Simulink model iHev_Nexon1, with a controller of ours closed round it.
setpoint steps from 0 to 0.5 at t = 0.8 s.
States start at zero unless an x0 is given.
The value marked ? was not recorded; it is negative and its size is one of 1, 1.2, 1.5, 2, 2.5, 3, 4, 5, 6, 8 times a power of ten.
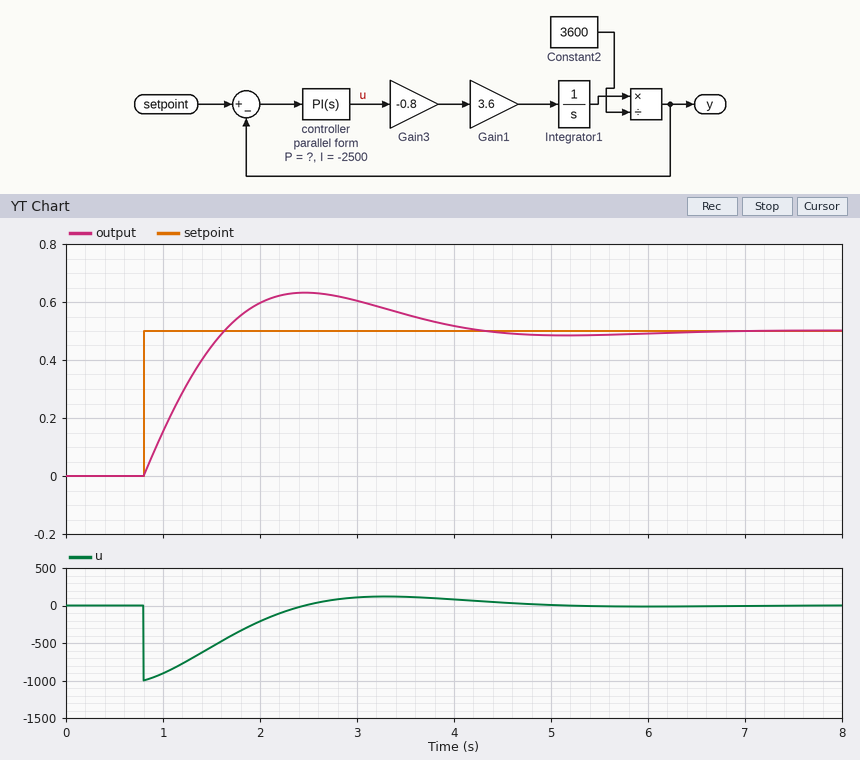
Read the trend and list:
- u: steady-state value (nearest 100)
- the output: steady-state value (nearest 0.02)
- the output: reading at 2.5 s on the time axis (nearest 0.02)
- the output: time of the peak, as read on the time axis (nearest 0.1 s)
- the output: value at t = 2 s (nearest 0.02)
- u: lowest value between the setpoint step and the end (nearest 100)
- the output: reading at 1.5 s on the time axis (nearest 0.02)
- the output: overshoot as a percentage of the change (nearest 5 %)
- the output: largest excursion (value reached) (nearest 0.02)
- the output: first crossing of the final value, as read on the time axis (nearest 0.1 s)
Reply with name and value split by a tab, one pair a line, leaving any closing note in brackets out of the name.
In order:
u: steady-state value	0
the output: steady-state value	0.50
the output: reading at 2.5 s on the time axis	0.64
the output: time of the peak, as read on the time axis	2.5 s
the output: value at t = 2 s	0.60
u: lowest value between the setpoint step and the end	-1000
the output: reading at 1.5 s on the time axis	0.44
the output: overshoot as a percentage of the change	25 %
the output: largest excursion (value reached)	0.64
the output: first crossing of the final value, as read on the time axis	1.6 s
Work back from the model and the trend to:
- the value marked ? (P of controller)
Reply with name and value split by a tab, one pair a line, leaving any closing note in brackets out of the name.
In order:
the value marked ?	-2000
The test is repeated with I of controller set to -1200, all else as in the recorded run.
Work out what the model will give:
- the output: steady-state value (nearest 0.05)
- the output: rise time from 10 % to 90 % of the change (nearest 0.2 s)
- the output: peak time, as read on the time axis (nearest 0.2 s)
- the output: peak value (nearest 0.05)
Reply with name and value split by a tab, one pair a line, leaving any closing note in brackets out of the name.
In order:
the output: steady-state value	0.50
the output: rise time from 10 % to 90 % of the change	0.8 s
the output: peak time, as read on the time axis	3.0 s
the output: peak value	0.60
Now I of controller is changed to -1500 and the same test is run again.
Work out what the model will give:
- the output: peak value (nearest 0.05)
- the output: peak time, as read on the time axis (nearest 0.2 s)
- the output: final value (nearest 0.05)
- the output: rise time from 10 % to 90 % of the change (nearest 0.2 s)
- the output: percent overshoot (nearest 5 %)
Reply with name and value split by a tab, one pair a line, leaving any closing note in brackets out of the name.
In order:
the output: peak value	0.60
the output: peak time, as read on the time axis	2.8 s
the output: final value	0.50
the output: rise time from 10 % to 90 % of the change	0.8 s
the output: percent overshoot	20 %
